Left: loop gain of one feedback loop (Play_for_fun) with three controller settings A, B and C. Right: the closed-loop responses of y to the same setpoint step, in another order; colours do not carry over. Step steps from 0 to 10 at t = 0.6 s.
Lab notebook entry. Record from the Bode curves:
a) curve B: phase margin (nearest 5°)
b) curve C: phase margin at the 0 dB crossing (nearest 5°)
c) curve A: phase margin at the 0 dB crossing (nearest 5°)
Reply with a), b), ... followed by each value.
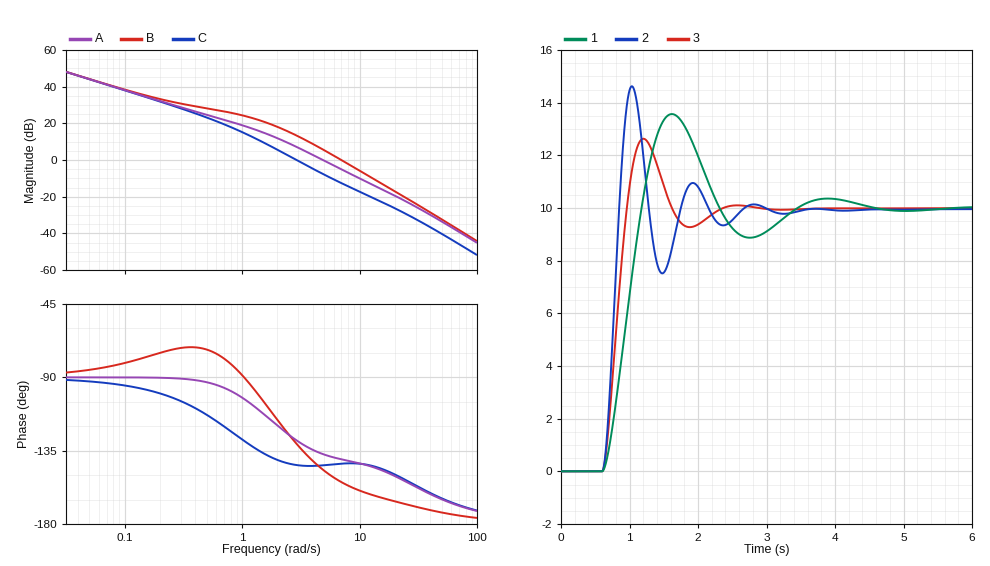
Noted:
a) 25°
b) 35°
c) 45°
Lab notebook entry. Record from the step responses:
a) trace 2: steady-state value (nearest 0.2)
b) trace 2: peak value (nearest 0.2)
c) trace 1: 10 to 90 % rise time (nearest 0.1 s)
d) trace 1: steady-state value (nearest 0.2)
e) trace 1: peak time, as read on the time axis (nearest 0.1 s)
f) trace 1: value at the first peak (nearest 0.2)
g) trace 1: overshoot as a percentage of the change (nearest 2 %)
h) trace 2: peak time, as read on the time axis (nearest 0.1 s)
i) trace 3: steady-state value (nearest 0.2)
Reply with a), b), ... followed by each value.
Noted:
a) 10.0
b) 14.6
c) 0.4 s
d) 10.0
e) 1.6 s
f) 13.6
g) 36 %
h) 1.0 s
i) 10.0
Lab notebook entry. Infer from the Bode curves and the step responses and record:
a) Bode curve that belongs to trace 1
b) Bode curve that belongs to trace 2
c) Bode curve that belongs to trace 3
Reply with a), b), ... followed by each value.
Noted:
a) C
b) B
c) A
